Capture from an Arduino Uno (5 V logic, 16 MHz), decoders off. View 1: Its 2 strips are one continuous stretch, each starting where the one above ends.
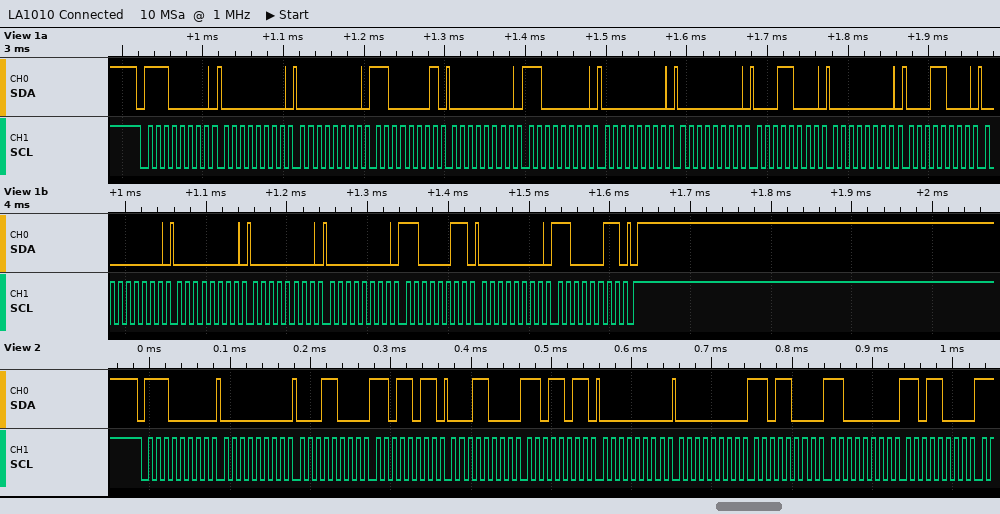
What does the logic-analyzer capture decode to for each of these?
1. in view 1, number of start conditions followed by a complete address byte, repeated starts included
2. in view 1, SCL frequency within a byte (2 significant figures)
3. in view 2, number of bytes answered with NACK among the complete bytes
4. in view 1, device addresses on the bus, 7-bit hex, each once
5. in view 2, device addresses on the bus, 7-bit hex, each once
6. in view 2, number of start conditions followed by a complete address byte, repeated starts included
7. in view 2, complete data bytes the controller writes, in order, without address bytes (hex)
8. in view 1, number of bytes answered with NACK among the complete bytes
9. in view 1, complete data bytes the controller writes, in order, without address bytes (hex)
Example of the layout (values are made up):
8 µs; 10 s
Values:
1; 100 kHz; 0; 0x70; 0x70; 1; 00 18 DB 18 DB 00 00 D8 C0 D8; 0; 00 00 C1 00 C0 00 00 18 00 18 00 00 00 00 C3 00 C3
